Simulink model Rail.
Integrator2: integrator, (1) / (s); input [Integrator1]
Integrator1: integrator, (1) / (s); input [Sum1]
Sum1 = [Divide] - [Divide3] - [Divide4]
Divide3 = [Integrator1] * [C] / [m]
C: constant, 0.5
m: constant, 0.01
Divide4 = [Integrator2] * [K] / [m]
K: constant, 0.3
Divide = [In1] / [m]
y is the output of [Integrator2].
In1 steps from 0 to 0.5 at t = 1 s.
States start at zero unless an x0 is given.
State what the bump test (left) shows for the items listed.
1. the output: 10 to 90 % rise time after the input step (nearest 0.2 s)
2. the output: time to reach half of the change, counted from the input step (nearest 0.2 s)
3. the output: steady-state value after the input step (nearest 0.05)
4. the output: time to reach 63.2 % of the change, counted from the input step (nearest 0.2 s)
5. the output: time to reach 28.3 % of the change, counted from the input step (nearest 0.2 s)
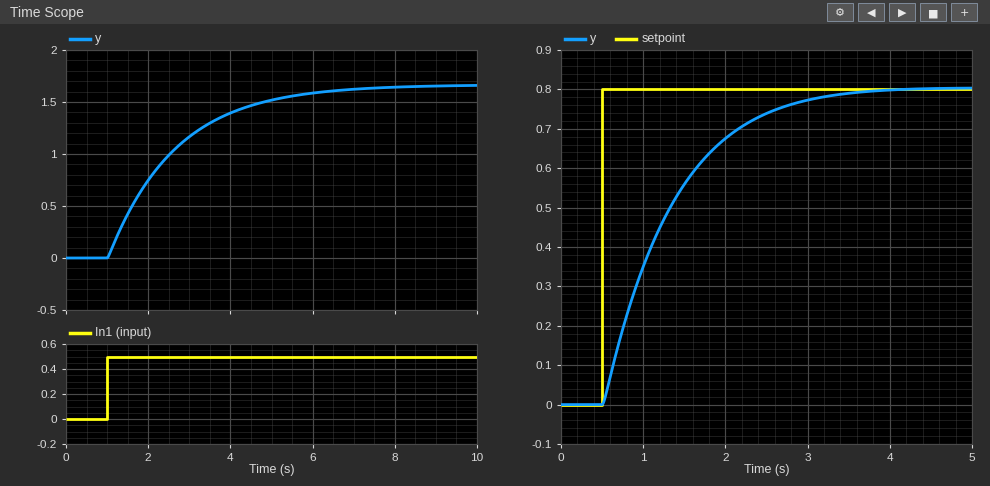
3.6 s
1.2 s
1.65
1.6 s
0.6 s
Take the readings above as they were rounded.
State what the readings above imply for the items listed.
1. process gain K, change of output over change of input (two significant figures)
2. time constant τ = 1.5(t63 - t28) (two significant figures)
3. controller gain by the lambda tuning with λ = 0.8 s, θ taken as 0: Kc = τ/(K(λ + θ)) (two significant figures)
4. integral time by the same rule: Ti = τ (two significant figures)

3.3
1.5 s
0.57
1.5 s
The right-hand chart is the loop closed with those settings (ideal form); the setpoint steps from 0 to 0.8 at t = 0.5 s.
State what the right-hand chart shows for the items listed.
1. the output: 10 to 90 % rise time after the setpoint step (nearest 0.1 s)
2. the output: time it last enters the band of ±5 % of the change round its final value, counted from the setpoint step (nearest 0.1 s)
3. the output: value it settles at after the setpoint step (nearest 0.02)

1.7 s
2.3 s
0.80
